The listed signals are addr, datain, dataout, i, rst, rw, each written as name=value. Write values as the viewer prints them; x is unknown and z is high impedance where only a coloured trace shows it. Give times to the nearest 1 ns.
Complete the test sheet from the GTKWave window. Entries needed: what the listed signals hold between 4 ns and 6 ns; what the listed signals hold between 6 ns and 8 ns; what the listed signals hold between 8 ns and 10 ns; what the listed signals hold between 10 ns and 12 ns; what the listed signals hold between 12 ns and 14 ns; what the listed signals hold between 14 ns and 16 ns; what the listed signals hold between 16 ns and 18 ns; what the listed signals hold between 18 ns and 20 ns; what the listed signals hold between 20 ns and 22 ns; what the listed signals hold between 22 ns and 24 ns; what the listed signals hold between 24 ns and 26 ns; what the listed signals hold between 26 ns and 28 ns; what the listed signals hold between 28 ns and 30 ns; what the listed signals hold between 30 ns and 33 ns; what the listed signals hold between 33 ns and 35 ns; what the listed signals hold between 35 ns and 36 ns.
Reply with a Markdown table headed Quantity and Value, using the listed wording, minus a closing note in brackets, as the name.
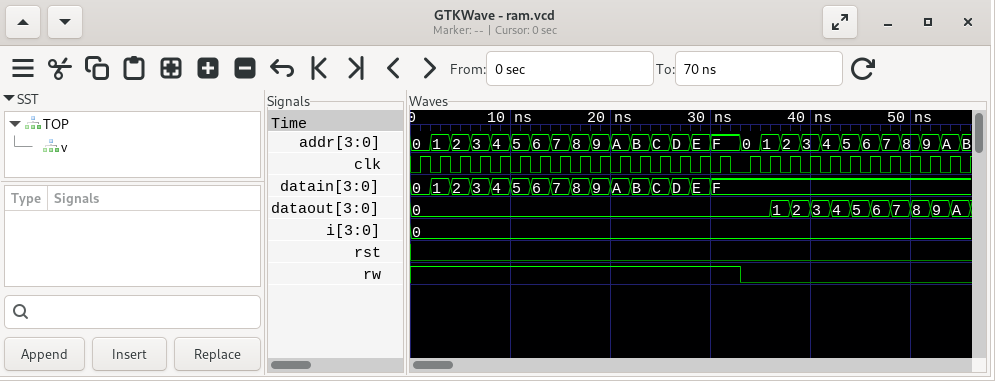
| Quantity | Value |
|---|---|
| what the listed signals hold between 4 ns and 6 ns | addr=2, datain=2, dataout=0, i=0, rst=0, rw=1 |
| what the listed signals hold between 6 ns and 8 ns | addr=3, datain=3, dataout=0, i=0, rst=0, rw=1 |
| what the listed signals hold between 8 ns and 10 ns | addr=4, datain=4, dataout=0, i=0, rst=0, rw=1 |
| what the listed signals hold between 10 ns and 12 ns | addr=5, datain=5, dataout=0, i=0, rst=0, rw=1 |
| what the listed signals hold between 12 ns and 14 ns | addr=6, datain=6, dataout=0, i=0, rst=0, rw=1 |
| what the listed signals hold between 14 ns and 16 ns | addr=7, datain=7, dataout=0, i=0, rst=0, rw=1 |
| what the listed signals hold between 16 ns and 18 ns | addr=8, datain=8, dataout=0, i=0, rst=0, rw=1 |
| what the listed signals hold between 18 ns and 20 ns | addr=9, datain=9, dataout=0, i=0, rst=0, rw=1 |
| what the listed signals hold between 20 ns and 22 ns | addr=A, datain=A, dataout=0, i=0, rst=0, rw=1 |
| what the listed signals hold between 22 ns and 24 ns | addr=B, datain=B, dataout=0, i=0, rst=0, rw=1 |
| what the listed signals hold between 24 ns and 26 ns | addr=C, datain=C, dataout=0, i=0, rst=0, rw=1 |
| what the listed signals hold between 26 ns and 28 ns | addr=D, datain=D, dataout=0, i=0, rst=0, rw=1 |
| what the listed signals hold between 28 ns and 30 ns | addr=E, datain=E, dataout=0, i=0, rst=0, rw=1 |
| what the listed signals hold between 30 ns and 33 ns | addr=F, datain=F, dataout=0, i=0, rst=0, rw=1 |
| what the listed signals hold between 33 ns and 35 ns | addr=0, datain=F, dataout=0, i=0, rst=0, rw=0 |
| what the listed signals hold between 35 ns and 36 ns | addr=1, datain=F, dataout=0, i=0, rst=0, rw=0 |
